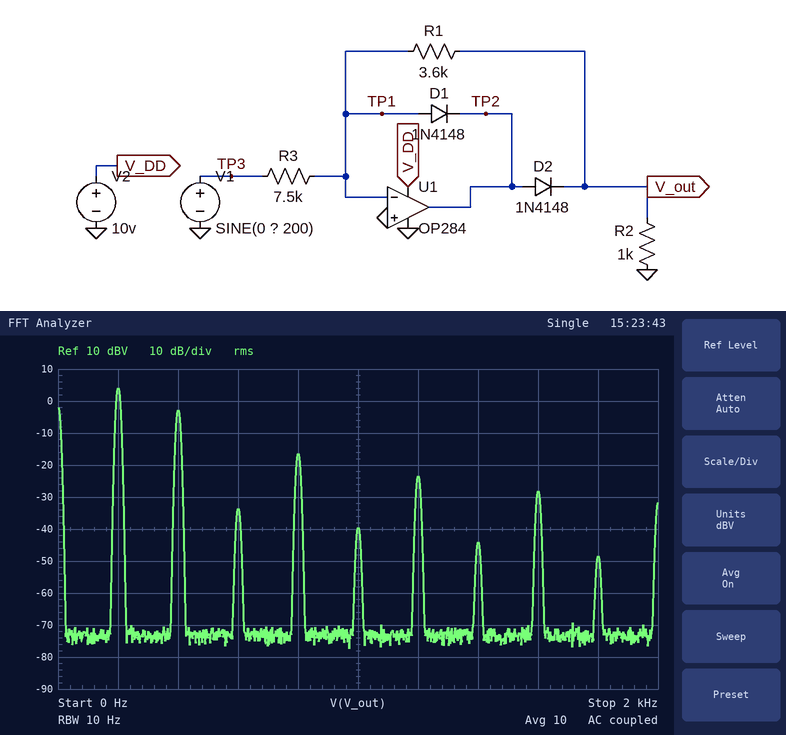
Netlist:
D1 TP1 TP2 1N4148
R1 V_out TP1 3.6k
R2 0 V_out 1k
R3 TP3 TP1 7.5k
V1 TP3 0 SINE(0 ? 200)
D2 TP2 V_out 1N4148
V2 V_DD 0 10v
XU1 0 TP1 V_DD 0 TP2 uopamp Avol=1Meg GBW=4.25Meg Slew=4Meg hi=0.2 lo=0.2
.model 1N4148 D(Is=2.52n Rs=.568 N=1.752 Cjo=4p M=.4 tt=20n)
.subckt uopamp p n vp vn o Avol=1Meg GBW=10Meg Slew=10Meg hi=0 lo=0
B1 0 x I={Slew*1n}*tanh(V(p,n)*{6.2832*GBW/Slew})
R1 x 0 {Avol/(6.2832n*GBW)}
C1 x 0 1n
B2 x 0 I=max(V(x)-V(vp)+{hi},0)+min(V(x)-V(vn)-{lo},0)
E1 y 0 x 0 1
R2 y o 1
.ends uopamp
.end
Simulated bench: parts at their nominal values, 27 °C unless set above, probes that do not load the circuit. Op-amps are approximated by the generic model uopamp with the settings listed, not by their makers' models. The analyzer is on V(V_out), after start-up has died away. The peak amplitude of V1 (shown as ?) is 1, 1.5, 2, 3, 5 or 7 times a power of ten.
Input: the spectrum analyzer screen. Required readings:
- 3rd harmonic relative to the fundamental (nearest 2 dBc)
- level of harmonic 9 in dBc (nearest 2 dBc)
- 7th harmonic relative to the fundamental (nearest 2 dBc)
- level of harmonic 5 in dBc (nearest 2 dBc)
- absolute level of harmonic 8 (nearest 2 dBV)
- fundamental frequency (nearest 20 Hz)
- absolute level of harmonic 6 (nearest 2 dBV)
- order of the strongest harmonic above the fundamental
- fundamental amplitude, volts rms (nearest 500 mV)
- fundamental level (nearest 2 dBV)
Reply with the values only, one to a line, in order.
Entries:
-38 dBc
-52 dBc
-48 dBc
-44 dBc
-28 dBV
200 Hz
-24 dBV
2
1.5 V
4 dBV
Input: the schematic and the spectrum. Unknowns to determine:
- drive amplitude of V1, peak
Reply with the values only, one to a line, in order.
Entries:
10 V
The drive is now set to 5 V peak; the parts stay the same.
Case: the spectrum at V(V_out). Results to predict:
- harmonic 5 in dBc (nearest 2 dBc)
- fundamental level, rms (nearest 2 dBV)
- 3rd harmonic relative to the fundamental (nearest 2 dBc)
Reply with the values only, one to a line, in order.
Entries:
-42 dBc
-2 dBV
-34 dBc
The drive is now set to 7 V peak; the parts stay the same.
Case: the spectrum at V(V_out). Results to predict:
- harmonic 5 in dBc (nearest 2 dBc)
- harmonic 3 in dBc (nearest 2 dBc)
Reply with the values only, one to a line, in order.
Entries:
-42 dBc
-36 dBc
